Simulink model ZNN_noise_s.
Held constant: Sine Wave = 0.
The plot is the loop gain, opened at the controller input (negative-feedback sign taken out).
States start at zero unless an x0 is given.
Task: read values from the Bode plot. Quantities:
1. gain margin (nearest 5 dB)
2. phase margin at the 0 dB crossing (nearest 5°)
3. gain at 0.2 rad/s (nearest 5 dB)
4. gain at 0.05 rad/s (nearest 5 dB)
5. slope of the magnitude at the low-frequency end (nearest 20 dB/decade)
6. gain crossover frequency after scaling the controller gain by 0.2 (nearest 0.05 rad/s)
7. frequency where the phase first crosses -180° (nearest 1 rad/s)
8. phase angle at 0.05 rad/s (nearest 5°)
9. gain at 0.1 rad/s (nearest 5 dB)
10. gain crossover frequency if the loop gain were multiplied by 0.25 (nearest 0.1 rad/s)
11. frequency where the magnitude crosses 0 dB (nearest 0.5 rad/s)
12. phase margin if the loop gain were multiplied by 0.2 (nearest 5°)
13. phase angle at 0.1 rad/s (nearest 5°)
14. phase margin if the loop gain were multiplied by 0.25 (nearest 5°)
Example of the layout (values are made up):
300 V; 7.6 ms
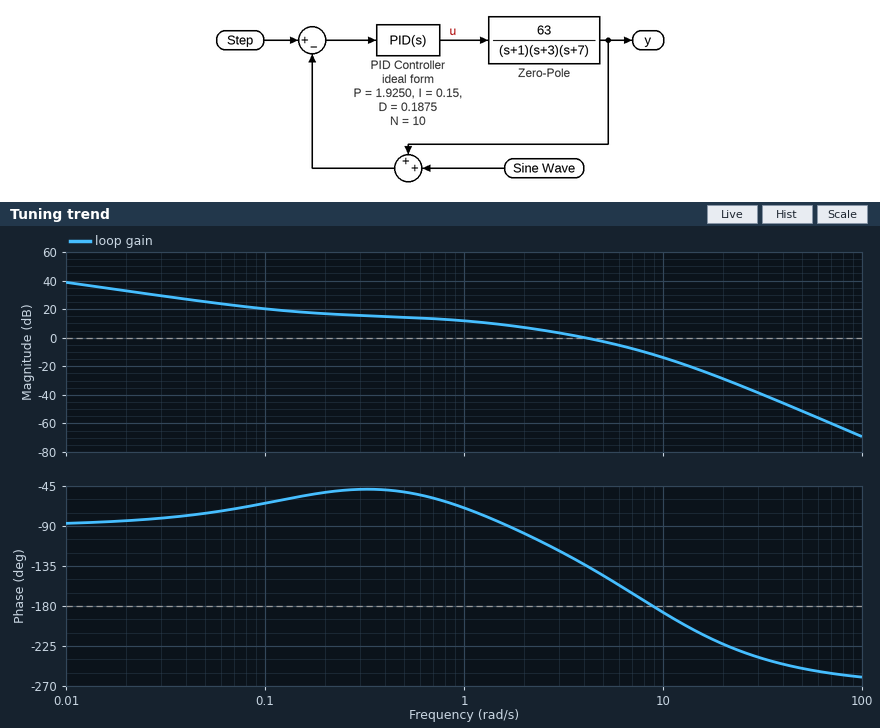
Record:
10 dB; 45°; 15 dB; 25 dB; -20 dB/decade; 0.55 rad/s; 9 rad/s; -75°; 20 dB; 1.0 rad/s; 4.0 rad/s; 125°; -65°; 110°
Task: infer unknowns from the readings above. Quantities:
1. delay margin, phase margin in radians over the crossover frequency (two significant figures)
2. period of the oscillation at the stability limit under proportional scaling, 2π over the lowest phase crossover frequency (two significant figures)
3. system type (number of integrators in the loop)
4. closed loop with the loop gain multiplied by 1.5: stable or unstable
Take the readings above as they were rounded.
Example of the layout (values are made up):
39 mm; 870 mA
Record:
0.20 s; 0.70 s; 1; stable
